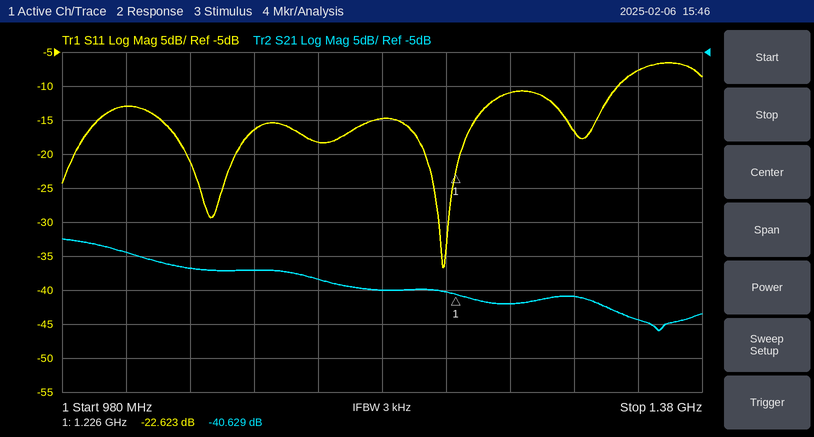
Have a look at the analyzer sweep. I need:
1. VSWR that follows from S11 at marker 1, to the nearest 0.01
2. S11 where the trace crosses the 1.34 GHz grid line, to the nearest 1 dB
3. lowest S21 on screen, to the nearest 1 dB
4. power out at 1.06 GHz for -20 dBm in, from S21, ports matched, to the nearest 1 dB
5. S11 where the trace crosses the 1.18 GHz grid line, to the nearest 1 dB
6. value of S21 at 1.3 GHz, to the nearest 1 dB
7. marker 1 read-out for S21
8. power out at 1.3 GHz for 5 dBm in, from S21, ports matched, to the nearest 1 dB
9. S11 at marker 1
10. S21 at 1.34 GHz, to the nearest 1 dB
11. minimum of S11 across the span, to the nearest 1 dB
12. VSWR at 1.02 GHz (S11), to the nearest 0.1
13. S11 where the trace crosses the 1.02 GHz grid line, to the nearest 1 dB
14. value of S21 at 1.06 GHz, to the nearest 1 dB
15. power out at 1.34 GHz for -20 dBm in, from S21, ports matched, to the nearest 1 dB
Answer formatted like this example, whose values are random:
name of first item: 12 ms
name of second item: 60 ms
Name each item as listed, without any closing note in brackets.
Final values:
VSWR that follows from S11 at marker 1, to the nearest 0.01: 1.16
S11 where the trace crosses the 1.34 GHz grid line, to the nearest 1 dB: -8 dB
lowest S21 on screen, to the nearest 1 dB: -46 dB
power out at 1.06 GHz for -20 dBm in, from S21, ports matched, to the nearest 1 dB: -57 dBm
S11 where the trace crosses the 1.18 GHz grid line, to the nearest 1 dB: -15 dB
value of S21 at 1.3 GHz, to the nearest 1 dB: -41 dB
marker 1 read-out for S21: -40.629 dB
power out at 1.3 GHz for 5 dBm in, from S21, ports matched, to the nearest 1 dB: -36 dBm
S11 at marker 1: -22.623 dB
S21 at 1.34 GHz, to the nearest 1 dB: -44 dB
minimum of S11 across the span, to the nearest 1 dB: -37 dB
VSWR at 1.02 GHz (S11), to the nearest 0.1: 1.6
S11 where the trace crosses the 1.02 GHz grid line, to the nearest 1 dB: -13 dB
value of S21 at 1.06 GHz, to the nearest 1 dB: -37 dB
power out at 1.34 GHz for -20 dBm in, from S21, ports matched, to the nearest 1 dB: -64 dBm
